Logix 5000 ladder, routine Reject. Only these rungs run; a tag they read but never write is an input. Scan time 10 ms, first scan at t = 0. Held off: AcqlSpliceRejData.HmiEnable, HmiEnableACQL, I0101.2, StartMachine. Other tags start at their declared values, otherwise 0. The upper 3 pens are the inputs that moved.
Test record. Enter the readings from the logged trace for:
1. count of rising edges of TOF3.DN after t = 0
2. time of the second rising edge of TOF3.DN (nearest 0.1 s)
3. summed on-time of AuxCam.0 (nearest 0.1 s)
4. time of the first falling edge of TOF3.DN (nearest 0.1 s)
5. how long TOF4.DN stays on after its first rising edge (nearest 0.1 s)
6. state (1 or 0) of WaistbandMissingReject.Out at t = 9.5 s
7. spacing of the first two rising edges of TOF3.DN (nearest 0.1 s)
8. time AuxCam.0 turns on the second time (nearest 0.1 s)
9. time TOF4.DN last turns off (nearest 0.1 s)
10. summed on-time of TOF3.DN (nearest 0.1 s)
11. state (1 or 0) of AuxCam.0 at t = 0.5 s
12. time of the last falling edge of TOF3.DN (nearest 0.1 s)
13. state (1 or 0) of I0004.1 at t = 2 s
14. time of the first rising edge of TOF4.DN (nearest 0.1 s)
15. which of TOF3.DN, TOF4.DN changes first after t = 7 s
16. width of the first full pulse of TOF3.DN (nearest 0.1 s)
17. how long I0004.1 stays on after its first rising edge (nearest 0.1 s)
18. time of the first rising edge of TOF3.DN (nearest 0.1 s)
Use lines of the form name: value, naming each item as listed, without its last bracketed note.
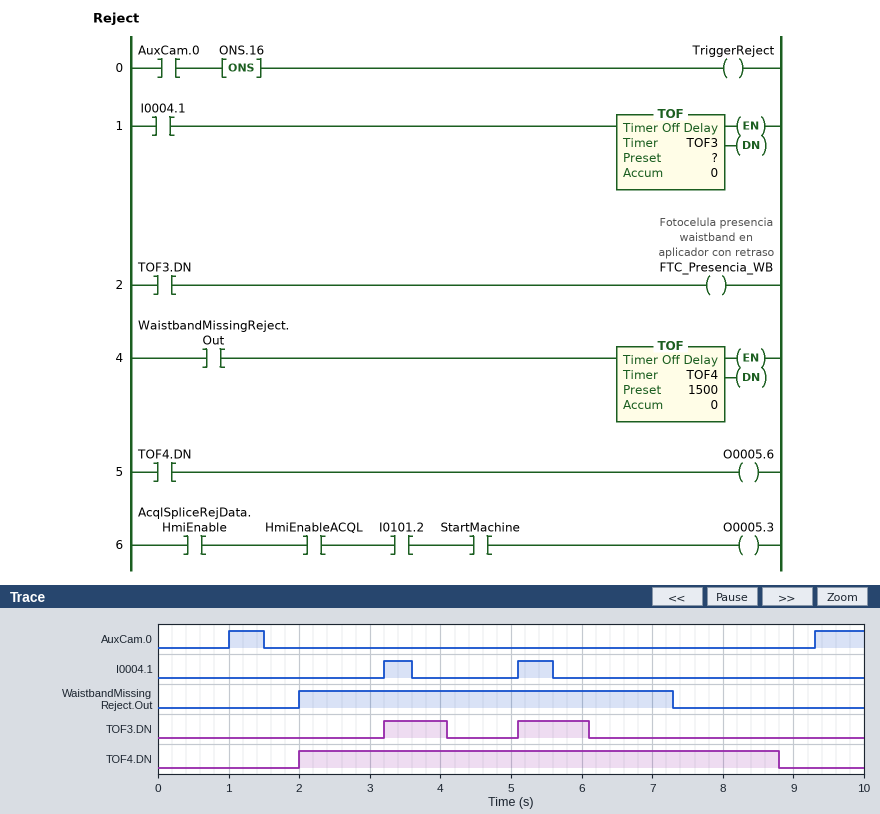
count of rising edges of TOF3.DN after t = 0: 2
time of the second rising edge of TOF3.DN: 5.1 s
summed on-time of AuxCam.0: 1.2 s
time of the first falling edge of TOF3.DN: 4.1 s
how long TOF4.DN stays on after its first rising edge: 6.8 s
state (1 or 0) of WaistbandMissingReject.Out at t = 9.5 s: 0
spacing of the first two rising edges of TOF3.DN: 1.9 s
time AuxCam.0 turns on the second time: 9.3 s
time TOF4.DN last turns off: 8.8 s
summed on-time of TOF3.DN: 1.9 s
state (1 or 0) of AuxCam.0 at t = 0.5 s: 0
time of the last falling edge of TOF3.DN: 6.1 s
state (1 or 0) of I0004.1 at t = 2 s: 0
time of the first rising edge of TOF4.DN: 2.0 s
which of TOF3.DN, TOF4.DN changes first after t = 7 s: TOF4.DN
width of the first full pulse of TOF3.DN: 0.9 s
how long I0004.1 stays on after its first rising edge: 0.4 s
time of the first rising edge of TOF3.DN: 3.2 s
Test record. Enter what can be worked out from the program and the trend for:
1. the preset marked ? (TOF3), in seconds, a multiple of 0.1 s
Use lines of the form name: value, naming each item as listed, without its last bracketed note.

the preset marked ? (TOF3), in seconds, a multiple of 0.1 s: 0.5 s
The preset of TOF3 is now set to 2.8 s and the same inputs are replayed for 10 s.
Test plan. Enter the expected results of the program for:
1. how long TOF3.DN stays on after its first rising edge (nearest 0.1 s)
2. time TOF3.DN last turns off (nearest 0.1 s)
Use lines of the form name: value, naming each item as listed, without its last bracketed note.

how long TOF3.DN stays on after its first rising edge: 5.2 s
time TOF3.DN last turns off: 8.4 s
